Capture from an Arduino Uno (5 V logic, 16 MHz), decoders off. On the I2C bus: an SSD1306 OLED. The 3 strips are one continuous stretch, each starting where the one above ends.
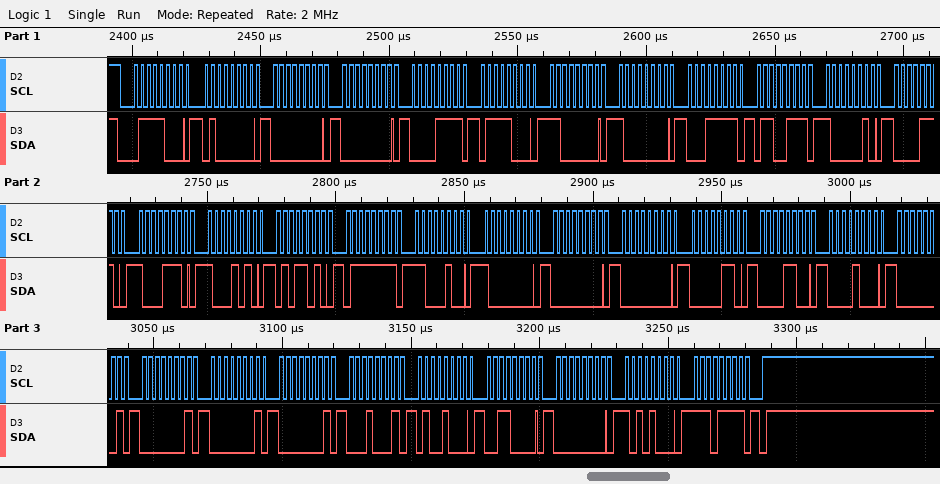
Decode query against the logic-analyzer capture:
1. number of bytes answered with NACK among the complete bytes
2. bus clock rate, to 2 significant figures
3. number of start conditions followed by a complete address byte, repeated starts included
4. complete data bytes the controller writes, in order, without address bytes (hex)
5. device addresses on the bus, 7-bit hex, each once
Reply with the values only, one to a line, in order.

0
400 kHz
1
40 00 00 0F 78 C0 80 1F 67 82 0E 8E 8A 5A 7F C4 80 00 00 06 0C 08 01 01 01 01 11 48 30 00 A8 EF
0x3C
